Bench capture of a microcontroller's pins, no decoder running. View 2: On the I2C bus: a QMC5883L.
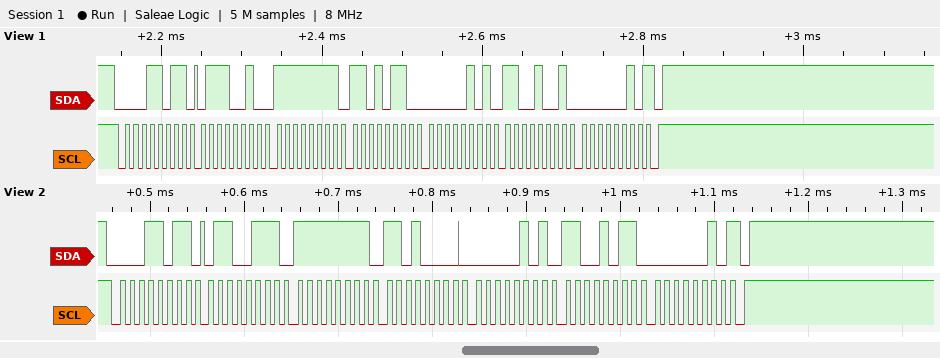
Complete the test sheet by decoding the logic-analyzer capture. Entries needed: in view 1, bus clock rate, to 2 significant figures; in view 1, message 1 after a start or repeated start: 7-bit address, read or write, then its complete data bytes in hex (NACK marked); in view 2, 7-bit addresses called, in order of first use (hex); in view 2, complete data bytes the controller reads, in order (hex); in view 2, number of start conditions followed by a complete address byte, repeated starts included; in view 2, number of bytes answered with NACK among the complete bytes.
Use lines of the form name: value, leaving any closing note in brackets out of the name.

in view 1, bus clock rate, to 2 significant figures: 100 kHz
in view 1, message 1 after a start or repeated start: 7-bit address, read or write, then its complete data bytes in hex: 0x0D read: 72 FF D6 05 C9 02 NACK
in view 2, 7-bit addresses called, in order of first use: 0x0D
in view 2, complete data bytes the controller reads, in order: 67 FF D0 05 CB 02
in view 2, number of start conditions followed by a complete address byte, repeated starts included: 1
in view 2, number of bytes answered with NACK among the complete bytes: 1
